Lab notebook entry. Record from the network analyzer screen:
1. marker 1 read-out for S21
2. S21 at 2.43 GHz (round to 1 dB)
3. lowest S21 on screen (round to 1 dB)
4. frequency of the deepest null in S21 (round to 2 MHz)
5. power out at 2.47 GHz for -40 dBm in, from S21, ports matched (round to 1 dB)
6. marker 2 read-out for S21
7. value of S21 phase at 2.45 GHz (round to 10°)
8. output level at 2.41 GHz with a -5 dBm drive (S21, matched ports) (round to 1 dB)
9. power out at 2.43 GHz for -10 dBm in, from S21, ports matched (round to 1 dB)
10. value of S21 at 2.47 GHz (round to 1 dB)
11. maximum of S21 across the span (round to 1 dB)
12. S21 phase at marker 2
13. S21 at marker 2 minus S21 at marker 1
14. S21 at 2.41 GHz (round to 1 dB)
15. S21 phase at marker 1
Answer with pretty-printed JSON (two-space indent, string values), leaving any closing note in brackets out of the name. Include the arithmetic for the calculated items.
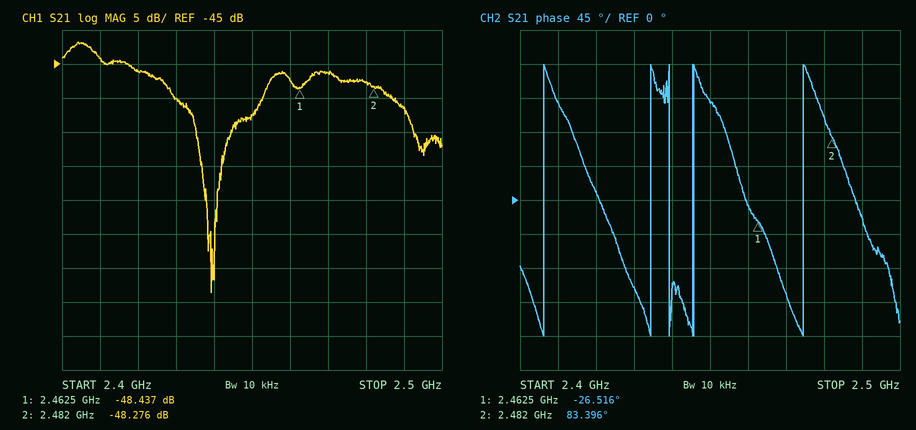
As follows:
{
  "marker 1 read-out for S21": "-48.437 dB",
  "S21 at 2.43 GHz": "-50 dB",
  "lowest S21 on screen": "-79 dB",
  "frequency of the deepest null in S21": "2.440 GHz",
  "power out at 2.47 GHz for -40 dBm in, from S21, ports matched": "-40 dBm + (-46 dB) = -86 dBm",
  "marker 2 read-out for S21": "-48.276 dB",
  "value of S21 phase at 2.45 GHz": "130°",
  "output level at 2.41 GHz with a -5 dBm drive (S21, matched ports)": "-5 dBm + (-44 dB) = -49 dBm",
  "power out at 2.43 GHz for -10 dBm in, from S21, ports matched": "-10 dBm + (-50 dB) = -60 dBm",
  "value of S21 at 2.47 GHz": "-46 dB",
  "maximum of S21 across the span": "-42 dB",
  "S21 phase at marker 2": "83.396°",
  "S21 at marker 2 minus S21 at marker 1": "-48.276 − (-48.437) = 0.161 dB",
  "S21 at 2.41 GHz": "-44 dB",
  "S21 phase at marker 1": "-26.516°"
}
